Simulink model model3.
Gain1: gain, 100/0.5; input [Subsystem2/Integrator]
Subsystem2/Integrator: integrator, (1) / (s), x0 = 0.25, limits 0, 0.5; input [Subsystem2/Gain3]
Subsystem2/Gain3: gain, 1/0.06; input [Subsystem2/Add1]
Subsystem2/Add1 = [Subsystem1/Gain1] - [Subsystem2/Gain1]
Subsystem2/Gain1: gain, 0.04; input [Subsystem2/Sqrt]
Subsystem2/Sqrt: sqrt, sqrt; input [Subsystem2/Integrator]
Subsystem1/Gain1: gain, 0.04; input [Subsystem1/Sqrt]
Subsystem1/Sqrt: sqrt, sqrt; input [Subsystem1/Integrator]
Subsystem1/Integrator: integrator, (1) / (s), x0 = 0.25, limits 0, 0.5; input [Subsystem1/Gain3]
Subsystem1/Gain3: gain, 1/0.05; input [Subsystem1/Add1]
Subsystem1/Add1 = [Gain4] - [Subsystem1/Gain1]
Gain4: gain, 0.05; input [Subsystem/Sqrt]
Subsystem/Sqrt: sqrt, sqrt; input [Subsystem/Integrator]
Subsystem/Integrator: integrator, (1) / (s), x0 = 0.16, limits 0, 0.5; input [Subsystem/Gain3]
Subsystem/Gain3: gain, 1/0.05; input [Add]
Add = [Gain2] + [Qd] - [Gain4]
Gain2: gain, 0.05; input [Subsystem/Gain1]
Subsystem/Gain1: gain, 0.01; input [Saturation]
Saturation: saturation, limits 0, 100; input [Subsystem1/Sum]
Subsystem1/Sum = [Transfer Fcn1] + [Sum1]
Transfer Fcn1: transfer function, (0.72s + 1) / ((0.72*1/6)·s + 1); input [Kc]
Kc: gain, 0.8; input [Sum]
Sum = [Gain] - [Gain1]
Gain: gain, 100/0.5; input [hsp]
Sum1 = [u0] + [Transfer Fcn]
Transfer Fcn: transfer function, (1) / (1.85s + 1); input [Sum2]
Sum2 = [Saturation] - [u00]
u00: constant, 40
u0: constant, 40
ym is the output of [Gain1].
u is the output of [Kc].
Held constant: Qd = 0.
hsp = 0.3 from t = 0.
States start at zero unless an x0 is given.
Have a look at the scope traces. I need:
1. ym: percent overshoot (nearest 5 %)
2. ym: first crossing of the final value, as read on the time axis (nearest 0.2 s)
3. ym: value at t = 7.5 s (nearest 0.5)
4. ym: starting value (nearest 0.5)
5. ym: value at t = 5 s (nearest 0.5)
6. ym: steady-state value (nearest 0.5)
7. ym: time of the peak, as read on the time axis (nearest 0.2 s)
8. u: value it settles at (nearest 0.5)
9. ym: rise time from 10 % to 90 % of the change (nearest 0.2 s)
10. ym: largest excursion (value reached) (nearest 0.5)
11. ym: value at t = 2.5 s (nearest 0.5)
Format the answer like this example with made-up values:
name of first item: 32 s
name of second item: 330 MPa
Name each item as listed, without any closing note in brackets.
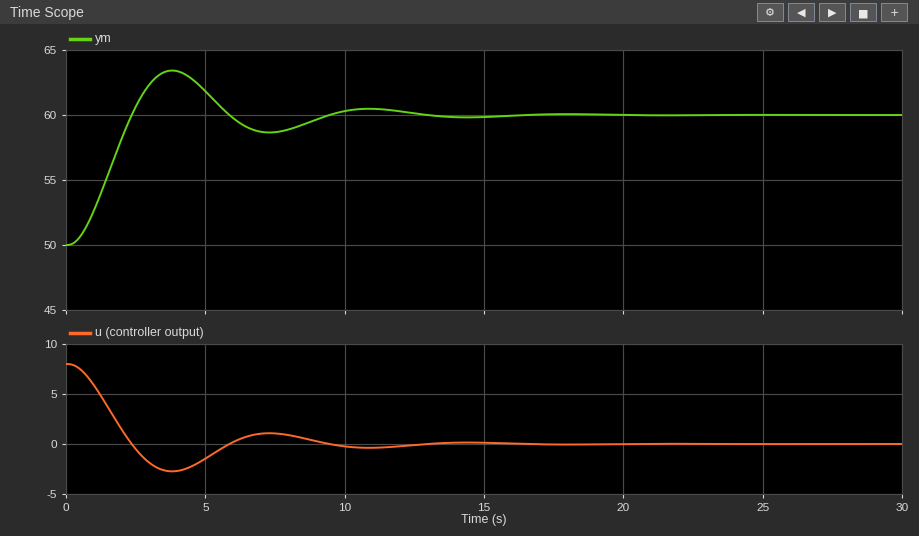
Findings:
ym: percent overshoot: 35 %
ym: first crossing of the final value, as read on the time axis: 2.4 s
ym: value at t = 7.5 s: 58.5
ym: starting value: 50.0
ym: value at t = 5 s: 62.0
ym: steady-state value: 60.0
ym: time of the peak, as read on the time axis: 3.8 s
u: value it settles at: 0.0
ym: rise time from 10 % to 90 % of the change: 1.6 s
ym: largest excursion (value reached): 63.5
ym: value at t = 2.5 s: 60.5
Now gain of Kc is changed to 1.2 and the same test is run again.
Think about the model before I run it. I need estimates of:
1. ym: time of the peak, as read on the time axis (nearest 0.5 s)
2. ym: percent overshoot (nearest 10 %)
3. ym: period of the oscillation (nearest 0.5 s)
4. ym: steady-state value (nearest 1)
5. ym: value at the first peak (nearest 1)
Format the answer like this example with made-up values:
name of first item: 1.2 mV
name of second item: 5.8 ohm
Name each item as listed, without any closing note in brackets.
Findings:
ym: time of the peak, as read on the time axis: 3.0 s
ym: percent overshoot: 50 %
ym: period of the oscillation: 5.5 s
ym: steady-state value: 60
ym: value at the first peak: 65
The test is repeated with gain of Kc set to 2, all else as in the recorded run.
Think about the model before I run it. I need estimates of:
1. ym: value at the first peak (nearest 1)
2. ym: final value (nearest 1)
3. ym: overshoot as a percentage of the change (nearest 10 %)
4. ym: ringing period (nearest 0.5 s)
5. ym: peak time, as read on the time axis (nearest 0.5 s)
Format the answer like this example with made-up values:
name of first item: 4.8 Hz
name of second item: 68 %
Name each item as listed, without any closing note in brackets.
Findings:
ym: value at the first peak: 66
ym: final value: 60
ym: overshoot as a percentage of the change: 60 %
ym: ringing period: 4.5 s
ym: peak time, as read on the time axis: 2.5 s
